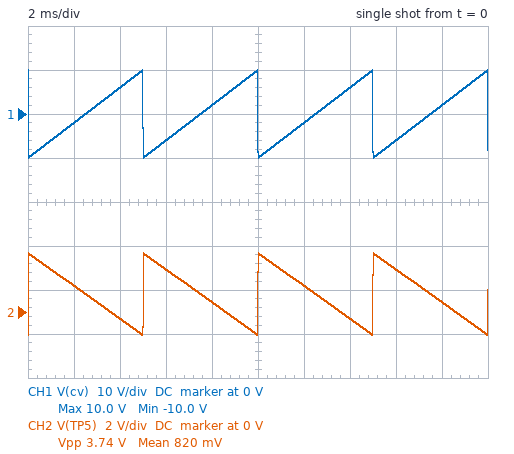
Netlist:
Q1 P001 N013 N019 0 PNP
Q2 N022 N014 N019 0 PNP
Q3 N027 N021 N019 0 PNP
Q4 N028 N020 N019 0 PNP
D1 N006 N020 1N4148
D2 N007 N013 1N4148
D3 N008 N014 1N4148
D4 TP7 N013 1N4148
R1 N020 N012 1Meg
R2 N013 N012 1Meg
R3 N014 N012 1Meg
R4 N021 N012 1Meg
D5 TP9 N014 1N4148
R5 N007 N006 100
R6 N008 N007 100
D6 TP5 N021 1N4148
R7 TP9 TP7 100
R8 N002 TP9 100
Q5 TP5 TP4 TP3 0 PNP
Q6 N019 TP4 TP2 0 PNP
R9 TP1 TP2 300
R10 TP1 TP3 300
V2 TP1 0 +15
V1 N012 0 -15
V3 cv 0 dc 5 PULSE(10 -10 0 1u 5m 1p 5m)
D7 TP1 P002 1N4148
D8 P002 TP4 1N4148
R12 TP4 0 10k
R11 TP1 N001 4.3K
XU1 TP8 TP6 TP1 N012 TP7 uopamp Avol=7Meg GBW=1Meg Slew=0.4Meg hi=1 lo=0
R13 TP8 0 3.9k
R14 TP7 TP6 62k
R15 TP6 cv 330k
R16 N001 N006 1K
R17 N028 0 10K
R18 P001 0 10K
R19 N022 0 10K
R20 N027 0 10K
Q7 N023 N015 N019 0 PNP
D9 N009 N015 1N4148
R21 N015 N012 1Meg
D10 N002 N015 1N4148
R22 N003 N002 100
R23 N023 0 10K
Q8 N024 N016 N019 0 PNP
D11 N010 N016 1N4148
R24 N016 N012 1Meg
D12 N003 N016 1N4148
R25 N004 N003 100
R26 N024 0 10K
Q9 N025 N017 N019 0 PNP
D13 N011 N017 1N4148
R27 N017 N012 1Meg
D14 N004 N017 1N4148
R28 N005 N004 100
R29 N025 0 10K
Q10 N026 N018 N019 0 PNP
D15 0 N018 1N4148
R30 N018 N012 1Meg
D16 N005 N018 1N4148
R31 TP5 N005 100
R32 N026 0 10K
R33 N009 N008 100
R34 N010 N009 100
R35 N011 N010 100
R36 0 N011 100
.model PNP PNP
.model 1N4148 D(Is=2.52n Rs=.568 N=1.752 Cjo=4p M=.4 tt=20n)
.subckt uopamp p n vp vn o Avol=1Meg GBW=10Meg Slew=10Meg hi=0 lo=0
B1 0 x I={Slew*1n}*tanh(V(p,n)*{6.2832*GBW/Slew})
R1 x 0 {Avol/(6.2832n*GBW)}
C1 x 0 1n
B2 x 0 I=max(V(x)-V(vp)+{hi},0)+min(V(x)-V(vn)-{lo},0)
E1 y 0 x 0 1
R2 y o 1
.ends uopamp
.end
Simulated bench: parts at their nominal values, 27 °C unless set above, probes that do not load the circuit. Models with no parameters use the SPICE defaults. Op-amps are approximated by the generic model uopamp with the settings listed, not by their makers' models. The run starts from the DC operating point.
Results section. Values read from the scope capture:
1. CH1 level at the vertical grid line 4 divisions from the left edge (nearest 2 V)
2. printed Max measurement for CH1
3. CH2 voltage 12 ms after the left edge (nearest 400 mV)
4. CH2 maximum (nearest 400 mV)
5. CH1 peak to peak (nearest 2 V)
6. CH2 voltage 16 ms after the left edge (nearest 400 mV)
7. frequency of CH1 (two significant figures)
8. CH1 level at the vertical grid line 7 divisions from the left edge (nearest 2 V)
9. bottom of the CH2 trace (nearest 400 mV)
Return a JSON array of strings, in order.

["2 V", "10.0 V", "1.2 V", "2.8 V", "20 V", "2.0 V", "200 Hz", "6 V", "-1.2 V"]
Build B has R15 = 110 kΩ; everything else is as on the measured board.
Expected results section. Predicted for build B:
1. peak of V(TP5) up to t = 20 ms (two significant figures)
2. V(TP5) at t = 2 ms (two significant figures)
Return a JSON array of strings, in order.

["6.4 V", "1.9 V"]
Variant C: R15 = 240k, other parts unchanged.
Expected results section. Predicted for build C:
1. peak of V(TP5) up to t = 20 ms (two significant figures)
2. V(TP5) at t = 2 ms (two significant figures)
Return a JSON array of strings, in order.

["3.4 V", "1.3 V"]
